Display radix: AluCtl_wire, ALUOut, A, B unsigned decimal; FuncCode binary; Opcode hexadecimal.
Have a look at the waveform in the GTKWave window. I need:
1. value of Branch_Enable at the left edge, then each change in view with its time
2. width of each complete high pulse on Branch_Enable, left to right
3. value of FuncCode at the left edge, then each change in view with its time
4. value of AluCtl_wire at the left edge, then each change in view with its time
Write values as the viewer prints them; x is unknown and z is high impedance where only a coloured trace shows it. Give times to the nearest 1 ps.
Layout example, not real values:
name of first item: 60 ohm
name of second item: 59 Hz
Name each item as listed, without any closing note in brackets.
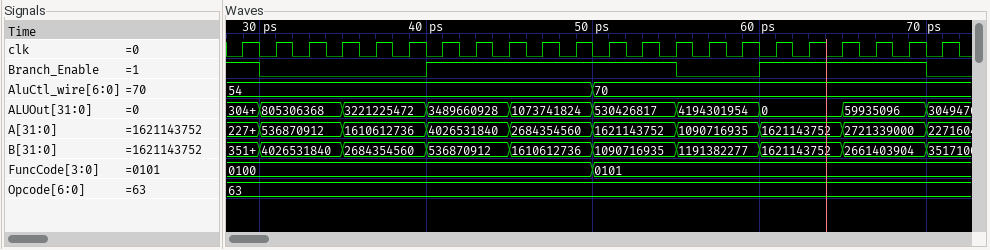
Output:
value of Branch_Enable at the left edge, then each change in view with its time: 1, 0 at 30 ps, 1 at 40 ps, 0 at 55 ps, 1 at 60 ps, 0 at 70 ps
width of each complete high pulse on Branch_Enable, left to right: 15 ps, 10 ps
value of FuncCode at the left edge, then each change in view with its time: 0100, 0101 at 50 ps
value of AluCtl_wire at the left edge, then each change in view with its time: 54, 70 at 50 ps
